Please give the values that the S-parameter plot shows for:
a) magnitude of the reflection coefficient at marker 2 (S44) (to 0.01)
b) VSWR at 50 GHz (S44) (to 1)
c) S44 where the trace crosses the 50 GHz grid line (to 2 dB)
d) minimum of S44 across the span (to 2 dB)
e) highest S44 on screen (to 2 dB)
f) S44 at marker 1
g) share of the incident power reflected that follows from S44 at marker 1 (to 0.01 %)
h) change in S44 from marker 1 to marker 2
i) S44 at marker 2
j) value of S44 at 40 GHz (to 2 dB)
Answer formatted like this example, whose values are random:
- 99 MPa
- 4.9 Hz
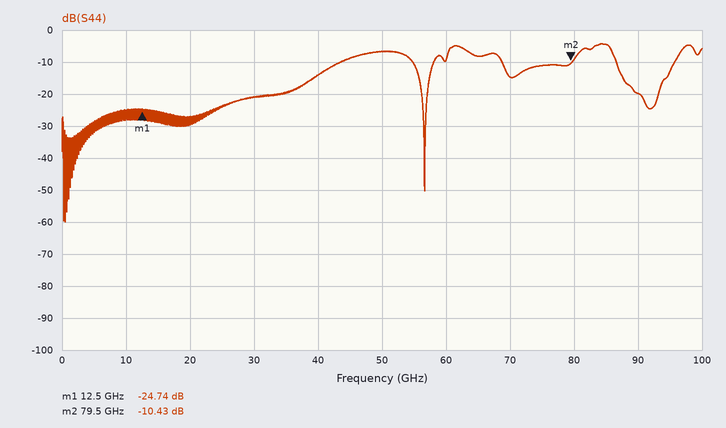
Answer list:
- 0.30
- 3
- -6 dB
- -60 dB
- -4 dB
- -24.74 dB
- 0.34 %
- 14.31 dB
- -10.43 dB
- -14 dB
